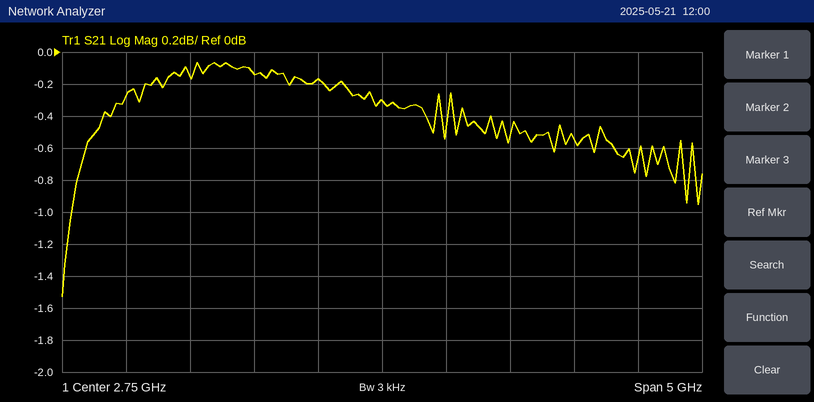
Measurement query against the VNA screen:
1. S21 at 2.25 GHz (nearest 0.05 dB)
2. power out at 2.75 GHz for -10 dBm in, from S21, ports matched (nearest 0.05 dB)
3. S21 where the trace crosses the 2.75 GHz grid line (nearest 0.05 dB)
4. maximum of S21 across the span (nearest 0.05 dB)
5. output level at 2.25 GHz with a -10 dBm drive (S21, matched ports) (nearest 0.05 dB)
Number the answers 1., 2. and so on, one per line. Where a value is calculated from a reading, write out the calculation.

1. -0.15 dB
2. -10 dBm + (-0.30 dB) = -10.30 dBm
3. -0.30 dB
4. -0.05 dB
5. -10 dBm + (-0.15 dB) = -10.15 dBm
